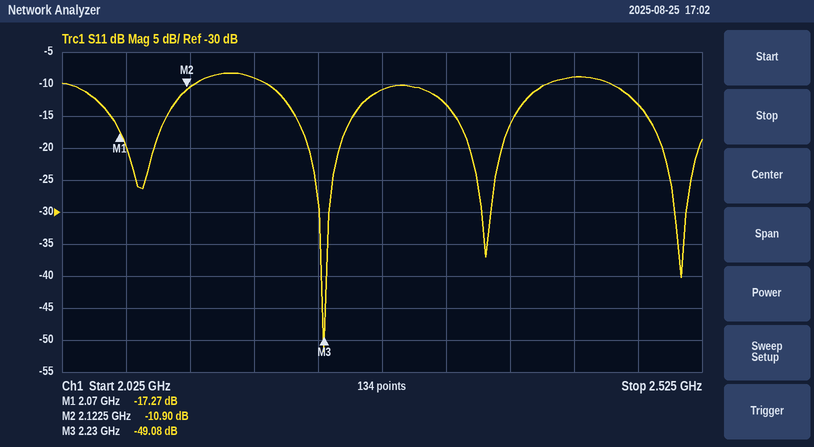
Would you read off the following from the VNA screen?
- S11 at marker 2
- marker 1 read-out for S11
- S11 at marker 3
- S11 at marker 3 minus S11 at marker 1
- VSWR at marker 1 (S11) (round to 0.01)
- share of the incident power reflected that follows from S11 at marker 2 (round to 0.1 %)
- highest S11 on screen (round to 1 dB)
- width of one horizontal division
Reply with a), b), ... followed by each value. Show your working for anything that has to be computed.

a) -10.90 dB
b) -17.27 dB
c) -49.08 dB
d) -49.08 − (-17.27) = -31.81 dB
e) (1 + 0.1369)/(1 − 0.1369) ≈ 1.32
f) 10^(-10.9/10) ≈ 8.1 %
g) -8 dB
h) 50 MHz
